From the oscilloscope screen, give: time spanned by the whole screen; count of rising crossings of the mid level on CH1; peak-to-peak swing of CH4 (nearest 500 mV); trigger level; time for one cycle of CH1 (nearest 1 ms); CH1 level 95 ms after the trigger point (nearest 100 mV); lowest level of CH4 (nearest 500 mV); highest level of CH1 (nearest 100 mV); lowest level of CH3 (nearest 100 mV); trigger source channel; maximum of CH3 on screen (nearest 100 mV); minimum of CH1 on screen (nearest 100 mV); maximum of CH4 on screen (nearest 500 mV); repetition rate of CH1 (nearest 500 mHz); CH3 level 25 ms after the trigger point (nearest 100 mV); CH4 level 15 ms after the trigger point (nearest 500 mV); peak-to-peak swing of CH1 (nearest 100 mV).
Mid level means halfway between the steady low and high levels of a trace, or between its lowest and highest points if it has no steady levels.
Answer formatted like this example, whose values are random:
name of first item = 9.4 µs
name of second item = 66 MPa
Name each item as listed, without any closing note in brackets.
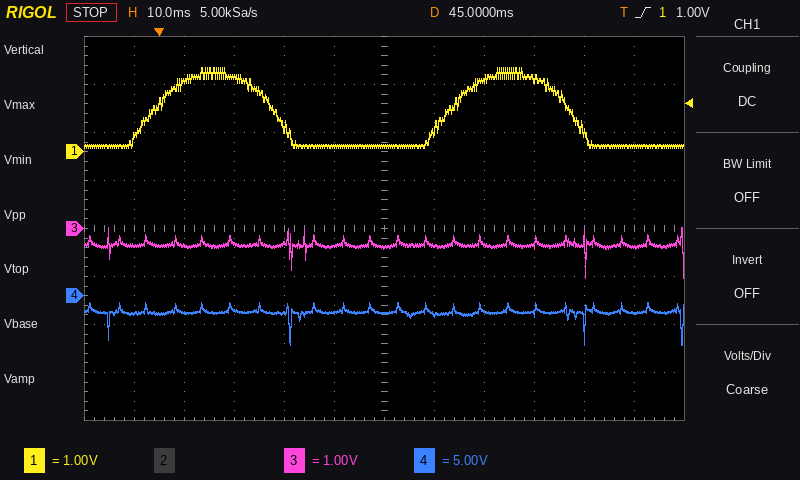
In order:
time spanned by the whole screen = 120 ms
count of rising crossings of the mid level on CH1 = 2
peak-to-peak swing of CH4 = 4.5 V
trigger level = 1.00 V
time for one cycle of CH1 = 59 ms
CH1 level 95 ms after the trigger point = 100 mV
lowest level of CH4 = -5.0 V
highest level of CH1 = 1.8 V
lowest level of CH3 = -1.0 V
trigger source channel = CH1
maximum of CH3 on screen = 0.0 V
minimum of CH1 on screen = 100 mV
maximum of CH4 on screen = -500 mV
repetition rate of CH1 = 17.0 Hz
CH3 level 25 ms after the trigger point = -300 mV
CH4 level 15 ms after the trigger point = -1.5 V
peak-to-peak swing of CH1 = 1.7 V
